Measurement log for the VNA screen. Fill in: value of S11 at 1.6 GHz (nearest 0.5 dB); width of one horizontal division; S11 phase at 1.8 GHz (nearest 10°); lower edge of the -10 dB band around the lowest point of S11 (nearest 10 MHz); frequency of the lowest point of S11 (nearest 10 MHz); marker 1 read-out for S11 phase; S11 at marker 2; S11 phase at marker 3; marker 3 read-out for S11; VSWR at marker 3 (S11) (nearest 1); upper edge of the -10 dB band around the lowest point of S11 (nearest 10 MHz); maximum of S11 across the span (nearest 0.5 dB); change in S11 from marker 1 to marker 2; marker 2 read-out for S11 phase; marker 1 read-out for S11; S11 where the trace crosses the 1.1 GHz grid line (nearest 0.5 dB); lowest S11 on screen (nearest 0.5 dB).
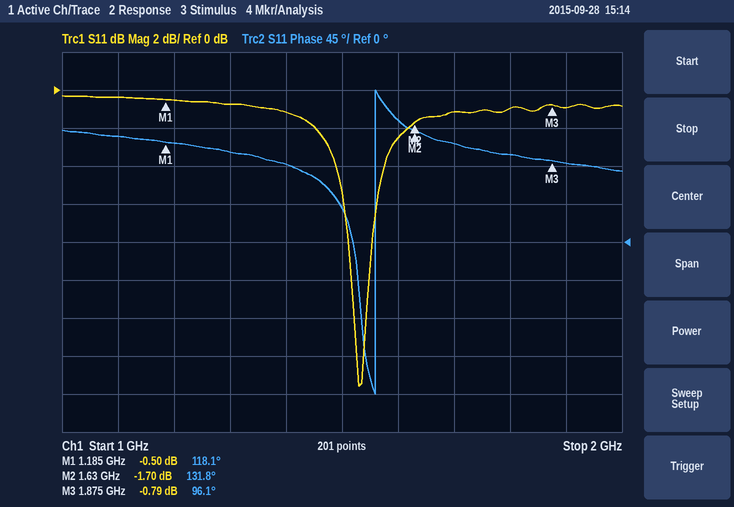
-2.5 dB
100 MHz
100°
1.52 GHz
1.53 GHz
118.1°
-1.70 dB
96.1°
-0.79 dB
22
1.55 GHz
-0.5 dB
-1.20 dB
131.8°
-0.50 dB
-0.5 dB
-15.5 dB
